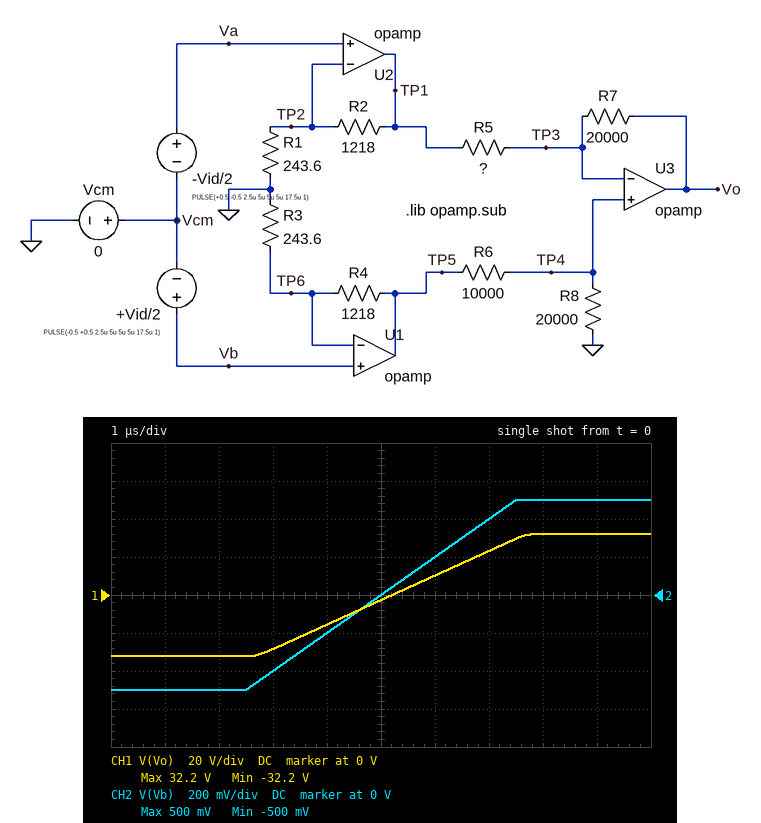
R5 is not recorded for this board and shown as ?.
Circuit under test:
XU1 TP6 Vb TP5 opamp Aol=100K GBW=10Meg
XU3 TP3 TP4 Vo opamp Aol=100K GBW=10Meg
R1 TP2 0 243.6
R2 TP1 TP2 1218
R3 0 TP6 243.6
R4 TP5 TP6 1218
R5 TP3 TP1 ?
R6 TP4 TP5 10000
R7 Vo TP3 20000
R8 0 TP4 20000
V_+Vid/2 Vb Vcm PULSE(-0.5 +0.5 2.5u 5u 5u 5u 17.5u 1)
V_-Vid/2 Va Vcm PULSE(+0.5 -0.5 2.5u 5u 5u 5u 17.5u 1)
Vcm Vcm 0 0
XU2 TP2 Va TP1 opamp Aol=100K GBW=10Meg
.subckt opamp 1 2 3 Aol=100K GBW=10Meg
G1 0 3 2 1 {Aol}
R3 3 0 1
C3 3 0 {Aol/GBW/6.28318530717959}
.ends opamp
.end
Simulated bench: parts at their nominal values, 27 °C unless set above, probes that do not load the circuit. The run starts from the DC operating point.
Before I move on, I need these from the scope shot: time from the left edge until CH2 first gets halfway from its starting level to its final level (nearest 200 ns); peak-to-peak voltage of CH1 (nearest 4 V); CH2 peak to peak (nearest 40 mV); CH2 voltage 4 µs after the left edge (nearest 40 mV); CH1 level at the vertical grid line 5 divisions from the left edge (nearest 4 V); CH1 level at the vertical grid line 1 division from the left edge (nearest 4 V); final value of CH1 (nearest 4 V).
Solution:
5.0 µs
64 V
1.00 V
-200 mV
-4 V
-32 V
32 V
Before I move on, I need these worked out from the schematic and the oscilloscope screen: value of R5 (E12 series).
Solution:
3.3 kΩ
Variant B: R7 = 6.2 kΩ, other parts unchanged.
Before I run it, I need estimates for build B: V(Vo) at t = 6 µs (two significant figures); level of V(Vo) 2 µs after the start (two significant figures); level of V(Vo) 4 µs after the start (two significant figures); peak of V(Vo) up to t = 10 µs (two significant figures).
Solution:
3.9 V
-11 V
-5.2 V
11 V
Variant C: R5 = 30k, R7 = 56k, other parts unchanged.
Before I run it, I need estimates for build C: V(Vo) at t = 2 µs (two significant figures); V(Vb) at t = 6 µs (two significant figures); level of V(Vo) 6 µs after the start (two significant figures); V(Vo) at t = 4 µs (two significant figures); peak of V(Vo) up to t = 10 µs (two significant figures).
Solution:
-11 V
200 mV
3.9 V
-5.2 V
11 V
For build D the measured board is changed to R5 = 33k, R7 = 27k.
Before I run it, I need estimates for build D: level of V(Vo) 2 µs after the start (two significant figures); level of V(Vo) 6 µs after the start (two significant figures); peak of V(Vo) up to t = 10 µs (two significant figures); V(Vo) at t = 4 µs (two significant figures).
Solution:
-6.1 V
2.1 V
6.1 V
-2.7 V
